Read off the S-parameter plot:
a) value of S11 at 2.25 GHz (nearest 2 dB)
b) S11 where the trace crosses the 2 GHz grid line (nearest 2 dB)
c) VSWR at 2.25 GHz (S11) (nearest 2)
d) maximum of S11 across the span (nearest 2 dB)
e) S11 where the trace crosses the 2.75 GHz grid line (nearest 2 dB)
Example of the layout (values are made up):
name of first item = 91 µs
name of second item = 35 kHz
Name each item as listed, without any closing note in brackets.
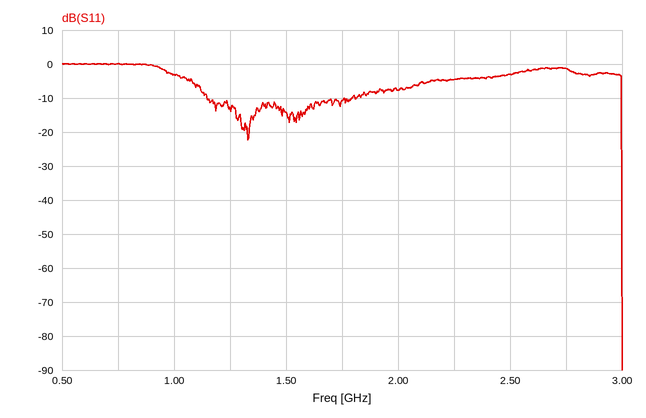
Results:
value of S11 at 2.25 GHz = -4 dB
S11 where the trace crosses the 2 GHz grid line = -8 dB
VSWR at 2.25 GHz (S11) = 4
maximum of S11 across the span = 0 dB
S11 where the trace crosses the 2.75 GHz grid line = -2 dB
